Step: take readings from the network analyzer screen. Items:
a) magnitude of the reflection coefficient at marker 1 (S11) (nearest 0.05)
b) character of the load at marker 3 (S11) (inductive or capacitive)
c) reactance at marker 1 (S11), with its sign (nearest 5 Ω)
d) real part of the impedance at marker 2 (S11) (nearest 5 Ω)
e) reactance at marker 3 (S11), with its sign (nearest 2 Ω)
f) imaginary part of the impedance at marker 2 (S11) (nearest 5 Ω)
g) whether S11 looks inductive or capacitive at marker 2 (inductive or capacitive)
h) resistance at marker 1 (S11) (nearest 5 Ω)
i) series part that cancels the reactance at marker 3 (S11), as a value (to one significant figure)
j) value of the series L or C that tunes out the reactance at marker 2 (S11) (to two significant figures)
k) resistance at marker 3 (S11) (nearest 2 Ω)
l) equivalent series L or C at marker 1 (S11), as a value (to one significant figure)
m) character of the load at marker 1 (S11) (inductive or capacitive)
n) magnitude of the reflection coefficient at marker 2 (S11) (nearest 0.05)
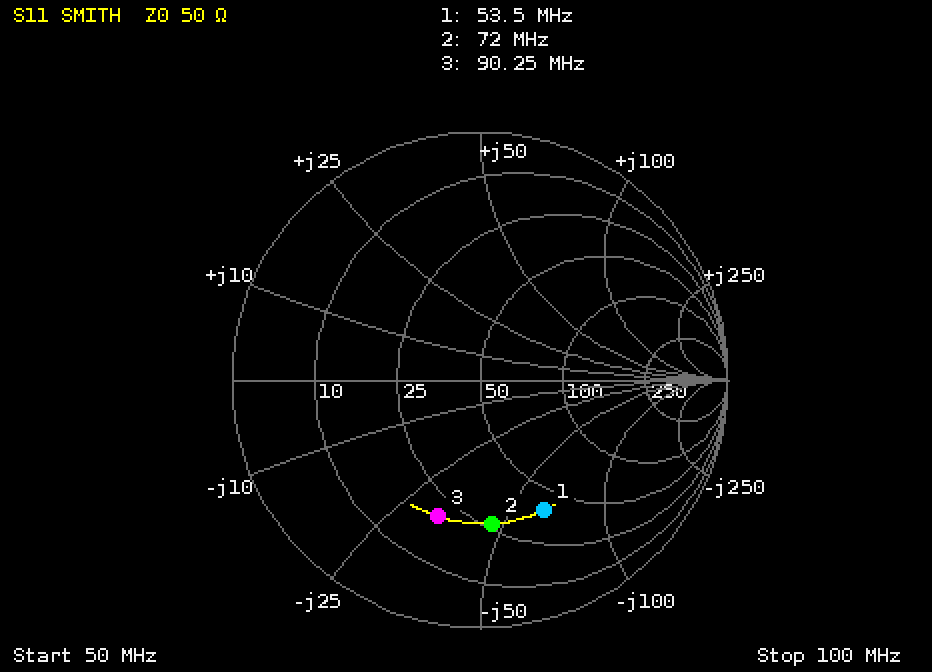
0.60
capacitive
-65 Ω
25 Ω
-32 Ω
-45 Ω
capacitive
40 Ω
60 nH
100 nH
20 Ω
50 pF
capacitive
0.60
